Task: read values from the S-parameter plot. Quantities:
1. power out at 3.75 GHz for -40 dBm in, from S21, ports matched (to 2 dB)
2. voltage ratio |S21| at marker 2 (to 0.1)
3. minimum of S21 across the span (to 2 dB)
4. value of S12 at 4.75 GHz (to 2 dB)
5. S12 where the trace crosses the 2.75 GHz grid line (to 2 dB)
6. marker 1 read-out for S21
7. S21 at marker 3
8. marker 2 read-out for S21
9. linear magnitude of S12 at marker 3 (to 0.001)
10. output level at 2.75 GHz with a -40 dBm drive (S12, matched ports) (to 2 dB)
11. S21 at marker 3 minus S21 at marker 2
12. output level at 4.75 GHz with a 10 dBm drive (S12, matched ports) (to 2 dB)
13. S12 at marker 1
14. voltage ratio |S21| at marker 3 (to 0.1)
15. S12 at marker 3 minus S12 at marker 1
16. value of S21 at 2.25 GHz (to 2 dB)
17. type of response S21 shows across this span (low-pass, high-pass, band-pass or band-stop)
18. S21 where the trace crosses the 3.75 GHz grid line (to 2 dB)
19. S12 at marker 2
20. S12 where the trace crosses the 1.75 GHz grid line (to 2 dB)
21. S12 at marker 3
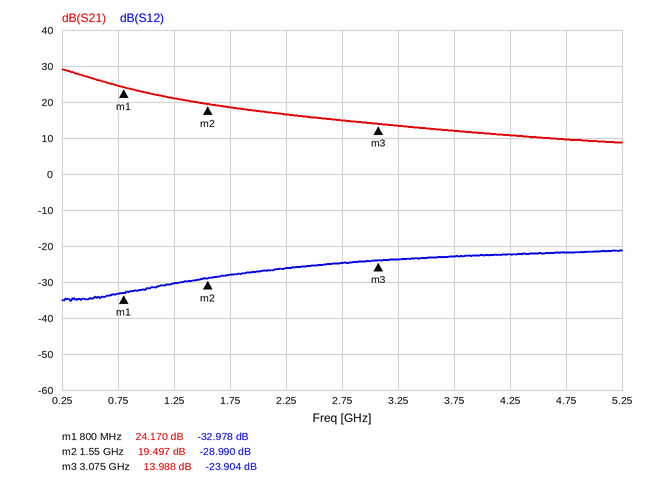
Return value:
-28 dBm
9.4
8 dB
-22 dB
-24 dB
24.170 dB
13.988 dB
19.497 dB
0.064
-64 dBm
-5.509 dB
-12 dBm
-32.978 dB
5.0
9.074 dB
16 dB
low-pass
12 dB
-28.990 dB
-28 dB
-23.904 dB
